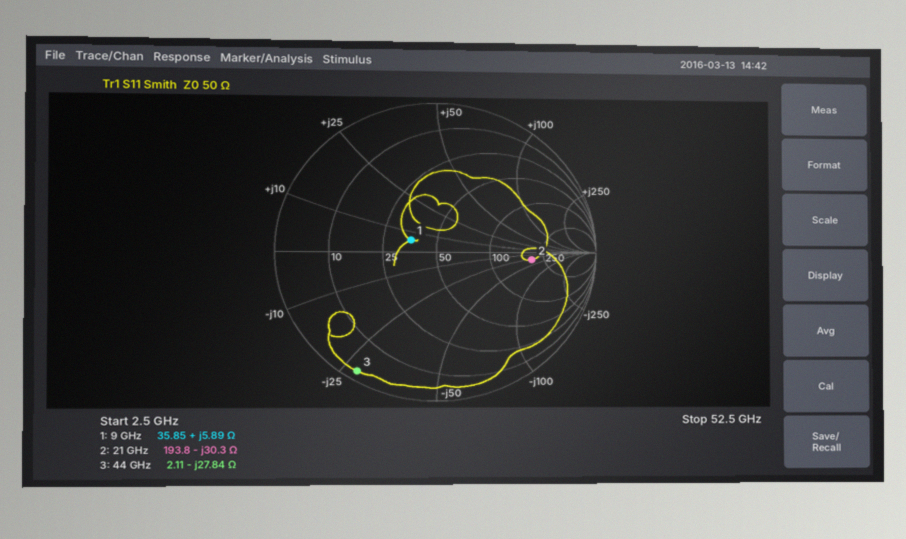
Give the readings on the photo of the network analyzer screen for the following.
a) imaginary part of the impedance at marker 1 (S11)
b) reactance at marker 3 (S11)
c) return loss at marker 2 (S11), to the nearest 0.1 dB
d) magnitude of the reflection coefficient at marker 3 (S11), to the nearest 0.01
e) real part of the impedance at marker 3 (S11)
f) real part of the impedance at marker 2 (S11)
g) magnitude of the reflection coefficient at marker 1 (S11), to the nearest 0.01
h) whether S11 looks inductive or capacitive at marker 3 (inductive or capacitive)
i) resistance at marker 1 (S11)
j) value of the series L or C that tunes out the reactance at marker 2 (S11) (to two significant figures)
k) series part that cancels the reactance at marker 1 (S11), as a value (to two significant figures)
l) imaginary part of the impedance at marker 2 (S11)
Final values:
+5.89 Ω
-27.84 Ω
4.5 dB
0.94
2.11 Ω
193.8 Ω
0.18
capacitive
35.85 Ω
230 pH
3.0 pF
-30.3 Ω
